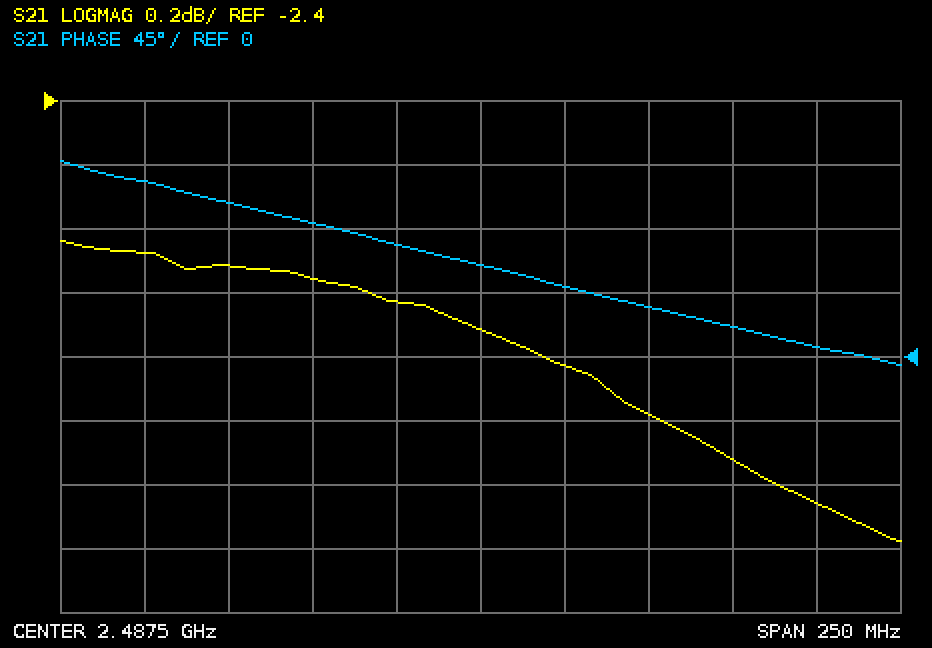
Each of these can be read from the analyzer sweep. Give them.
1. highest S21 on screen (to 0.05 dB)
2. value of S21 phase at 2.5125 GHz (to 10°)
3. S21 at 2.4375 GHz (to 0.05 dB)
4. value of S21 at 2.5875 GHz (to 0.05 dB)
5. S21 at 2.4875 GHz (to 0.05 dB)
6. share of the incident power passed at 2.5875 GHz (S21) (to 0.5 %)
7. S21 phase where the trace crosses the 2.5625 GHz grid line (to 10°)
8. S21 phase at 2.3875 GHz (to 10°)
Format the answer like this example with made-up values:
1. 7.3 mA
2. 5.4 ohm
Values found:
1. -2.85 dB
2. 50°
3. -2.95 dB
4. -3.65 dB
5. -3.10 dB
6. 43.0 %
7. 20°
8. 120°
